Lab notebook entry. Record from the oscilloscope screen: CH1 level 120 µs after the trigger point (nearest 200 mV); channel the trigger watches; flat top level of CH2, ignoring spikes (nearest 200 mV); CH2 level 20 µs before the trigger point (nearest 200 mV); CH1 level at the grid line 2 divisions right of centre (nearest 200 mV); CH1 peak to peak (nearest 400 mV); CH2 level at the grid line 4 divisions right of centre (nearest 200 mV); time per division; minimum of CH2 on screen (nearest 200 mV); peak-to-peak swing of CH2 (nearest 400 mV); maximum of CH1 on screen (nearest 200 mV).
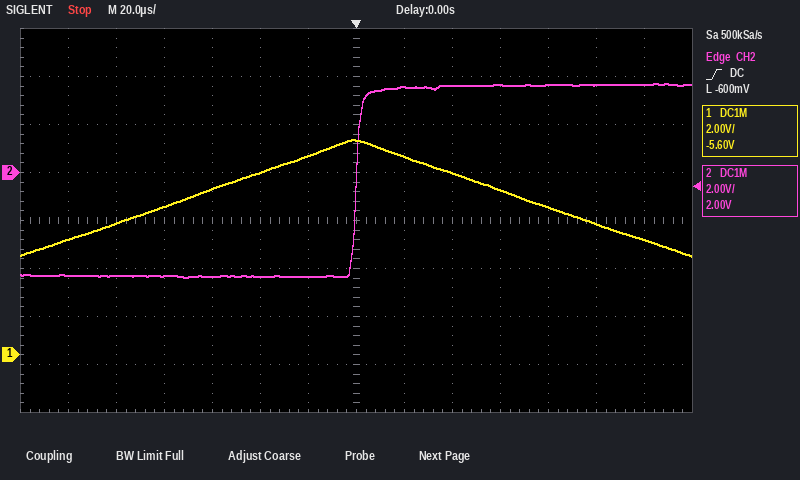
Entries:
4.8 V
CH2
3.6 V
-4.4 V
7.6 V
4.8 V
3.6 V
20 µs
-4.4 V
8.0 V
9.0 V
